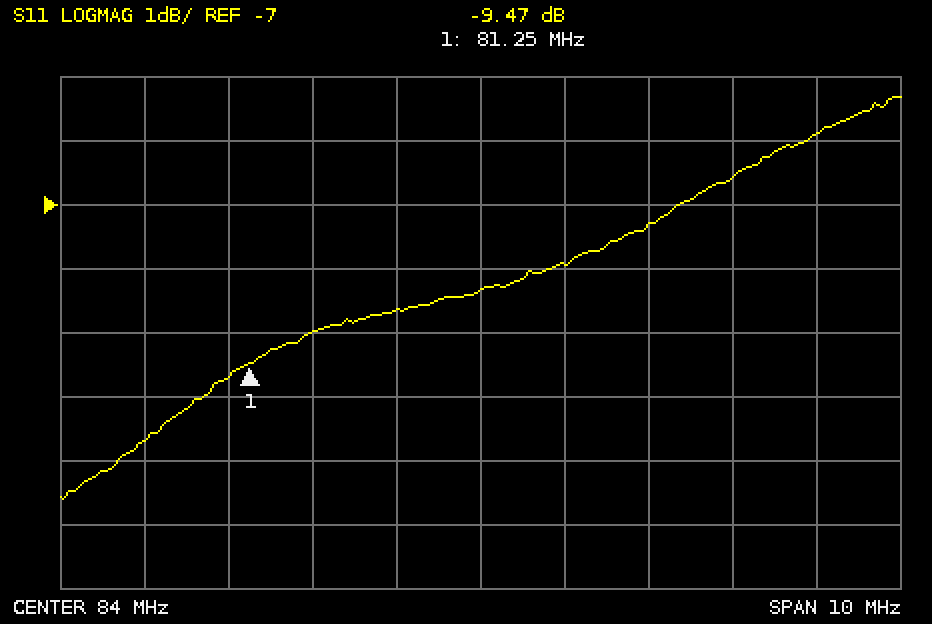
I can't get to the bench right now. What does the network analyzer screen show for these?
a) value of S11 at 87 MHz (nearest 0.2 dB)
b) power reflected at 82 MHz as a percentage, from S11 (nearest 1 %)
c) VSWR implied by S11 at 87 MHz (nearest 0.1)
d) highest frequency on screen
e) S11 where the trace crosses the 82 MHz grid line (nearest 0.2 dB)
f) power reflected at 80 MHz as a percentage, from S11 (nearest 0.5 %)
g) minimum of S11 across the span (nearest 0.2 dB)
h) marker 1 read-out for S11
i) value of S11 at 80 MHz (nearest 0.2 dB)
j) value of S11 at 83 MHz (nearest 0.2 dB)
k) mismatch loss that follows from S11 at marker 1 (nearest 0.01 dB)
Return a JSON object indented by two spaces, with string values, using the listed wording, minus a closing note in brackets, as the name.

{
  "value of S11 at 87 MHz": "-6.6 dB",
  "power reflected at 82 MHz as a percentage, from S11": "13 %",
  "VSWR implied by S11 at 87 MHz": "2.8",
  "highest frequency on screen": "89 MHz",
  "S11 where the trace crosses the 82 MHz grid line": "-9.0 dB",
  "power reflected at 80 MHz as a percentage, from S11": "8.5 %",
  "minimum of S11 across the span": "-11.6 dB",
  "marker 1 read-out for S11": "-9.47 dB",
  "value of S11 at 80 MHz": "-10.6 dB",
  "value of S11 at 83 MHz": "-8.6 dB",
  "mismatch loss that follows from S11 at marker 1": "0.52 dB"
}
